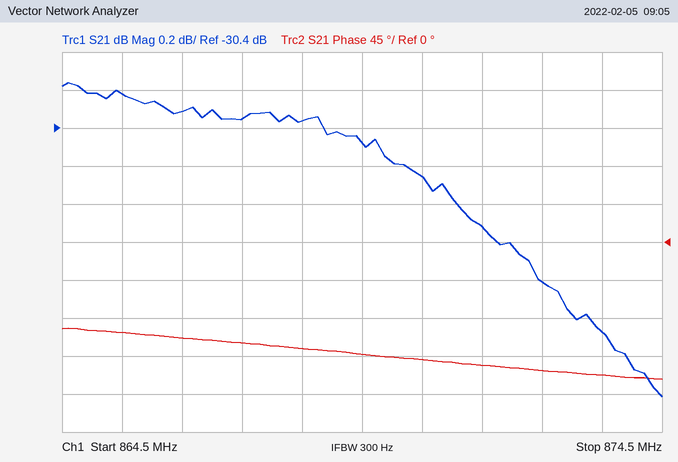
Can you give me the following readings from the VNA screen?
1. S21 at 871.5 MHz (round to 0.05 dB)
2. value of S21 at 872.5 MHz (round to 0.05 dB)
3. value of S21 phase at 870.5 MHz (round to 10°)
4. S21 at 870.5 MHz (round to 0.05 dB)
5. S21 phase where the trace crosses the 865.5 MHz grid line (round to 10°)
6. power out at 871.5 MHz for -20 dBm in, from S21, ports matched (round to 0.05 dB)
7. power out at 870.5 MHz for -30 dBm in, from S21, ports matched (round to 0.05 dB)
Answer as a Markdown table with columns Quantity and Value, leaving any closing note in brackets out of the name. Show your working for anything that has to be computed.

| Quantity | Value |
|---|---|
| S21 at 871.5 MHz | -30.90 dB |
| value of S21 at 872.5 MHz | -31.20 dB |
| value of S21 phase at 870.5 MHz | -140° |
| S21 at 870.5 MHz | -30.65 dB |
| S21 phase where the trace crosses the 865.5 MHz grid line | -110° |
| power out at 871.5 MHz for -20 dBm in, from S21, ports matched | -20 dBm + (-30.90 dB) = -50.90 dBm |
| power out at 870.5 MHz for -30 dBm in, from S21, ports matched | -30 dBm + (-30.65 dB) = -60.65 dBm |
